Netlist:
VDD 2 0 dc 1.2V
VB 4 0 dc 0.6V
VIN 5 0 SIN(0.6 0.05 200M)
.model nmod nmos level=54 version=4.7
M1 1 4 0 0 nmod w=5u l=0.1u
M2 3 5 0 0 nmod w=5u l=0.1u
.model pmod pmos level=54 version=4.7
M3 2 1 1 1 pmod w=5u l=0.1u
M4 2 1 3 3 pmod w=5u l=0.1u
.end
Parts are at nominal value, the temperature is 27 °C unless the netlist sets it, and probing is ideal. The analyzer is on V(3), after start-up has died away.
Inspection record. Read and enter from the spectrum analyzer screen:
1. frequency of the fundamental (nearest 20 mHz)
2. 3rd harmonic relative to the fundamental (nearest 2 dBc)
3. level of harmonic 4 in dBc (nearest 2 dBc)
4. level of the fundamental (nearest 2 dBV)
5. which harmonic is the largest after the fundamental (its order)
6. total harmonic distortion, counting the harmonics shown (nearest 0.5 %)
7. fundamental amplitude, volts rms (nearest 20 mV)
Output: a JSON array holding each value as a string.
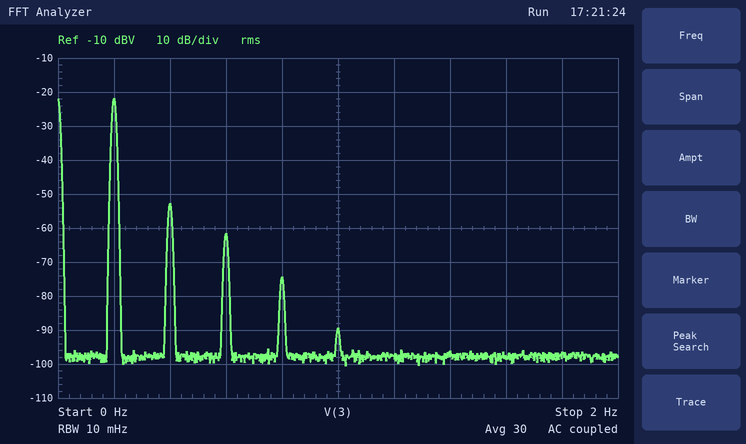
["200 mHz", "-40 dBc", "-52 dBc", "-22 dBV", "2", "3.0 %", "80 mV"]
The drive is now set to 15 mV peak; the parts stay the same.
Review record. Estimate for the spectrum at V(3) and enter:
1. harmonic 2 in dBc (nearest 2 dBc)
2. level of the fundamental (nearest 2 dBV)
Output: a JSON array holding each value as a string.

["-38 dBc", "-32 dBV"]
